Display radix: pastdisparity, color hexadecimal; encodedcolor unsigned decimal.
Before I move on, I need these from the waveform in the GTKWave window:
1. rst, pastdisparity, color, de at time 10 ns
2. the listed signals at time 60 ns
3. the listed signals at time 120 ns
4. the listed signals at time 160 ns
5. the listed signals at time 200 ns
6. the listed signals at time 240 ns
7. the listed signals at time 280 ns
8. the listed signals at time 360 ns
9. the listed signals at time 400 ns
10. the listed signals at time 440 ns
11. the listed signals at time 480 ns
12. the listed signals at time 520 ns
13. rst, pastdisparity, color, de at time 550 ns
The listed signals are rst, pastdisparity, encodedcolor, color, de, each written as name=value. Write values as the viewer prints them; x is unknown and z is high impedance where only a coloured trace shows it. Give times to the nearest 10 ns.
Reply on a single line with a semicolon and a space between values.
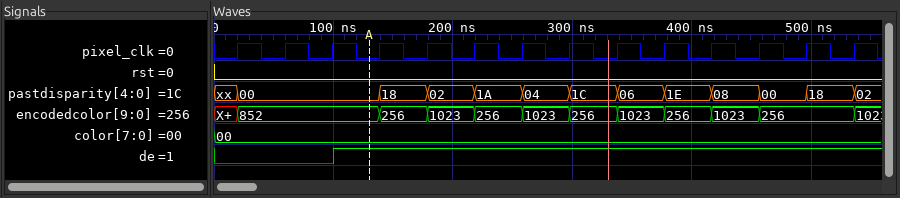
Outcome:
rst=0, pastdisparity=xx, color=00, de=0; rst=0, pastdisparity=00, encodedcolor=852, color=00, de=0; rst=0, pastdisparity=00, encodedcolor=852, color=00, de=1; rst=0, pastdisparity=18, encodedcolor=256, color=00, de=1; rst=0, pastdisparity=02, encodedcolor=1023, color=00, de=1; rst=0, pastdisparity=1A, encodedcolor=256, color=00, de=1; rst=0, pastdisparity=04, encodedcolor=1023, color=00, de=1; rst=0, pastdisparity=06, encodedcolor=1023, color=00, de=1; rst=0, pastdisparity=1E, encodedcolor=256, color=00, de=1; rst=0, pastdisparity=08, encodedcolor=1023, color=00, de=1; rst=0, pastdisparity=00, encodedcolor=256, color=00, de=1; rst=0, pastdisparity=18, encodedcolor=256, color=00, de=1; rst=0, pastdisparity=02, color=00, de=1
